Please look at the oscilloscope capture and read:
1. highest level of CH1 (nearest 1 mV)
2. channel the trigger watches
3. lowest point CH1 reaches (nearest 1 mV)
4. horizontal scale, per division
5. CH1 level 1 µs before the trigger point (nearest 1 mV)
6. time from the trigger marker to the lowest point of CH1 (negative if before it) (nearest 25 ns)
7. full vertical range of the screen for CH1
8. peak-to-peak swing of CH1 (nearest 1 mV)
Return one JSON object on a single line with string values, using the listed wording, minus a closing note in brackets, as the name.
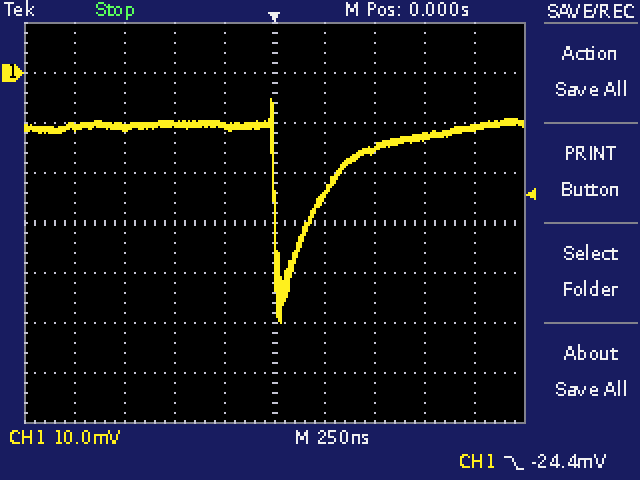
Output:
{"highest level of CH1": "-5 mV", "channel the trigger watches": "CH1", "lowest point CH1 reaches": "-50 mV", "horizontal scale, per division": "250 ns", "CH1 level 1 µs before the trigger point": "-11 mV", "time from the trigger marker to the lowest point of CH1 (negative if before it)": "+25 ns", "full vertical range of the screen for CH1": "80 mV", "peak-to-peak swing of CH1": "45 mV"}
